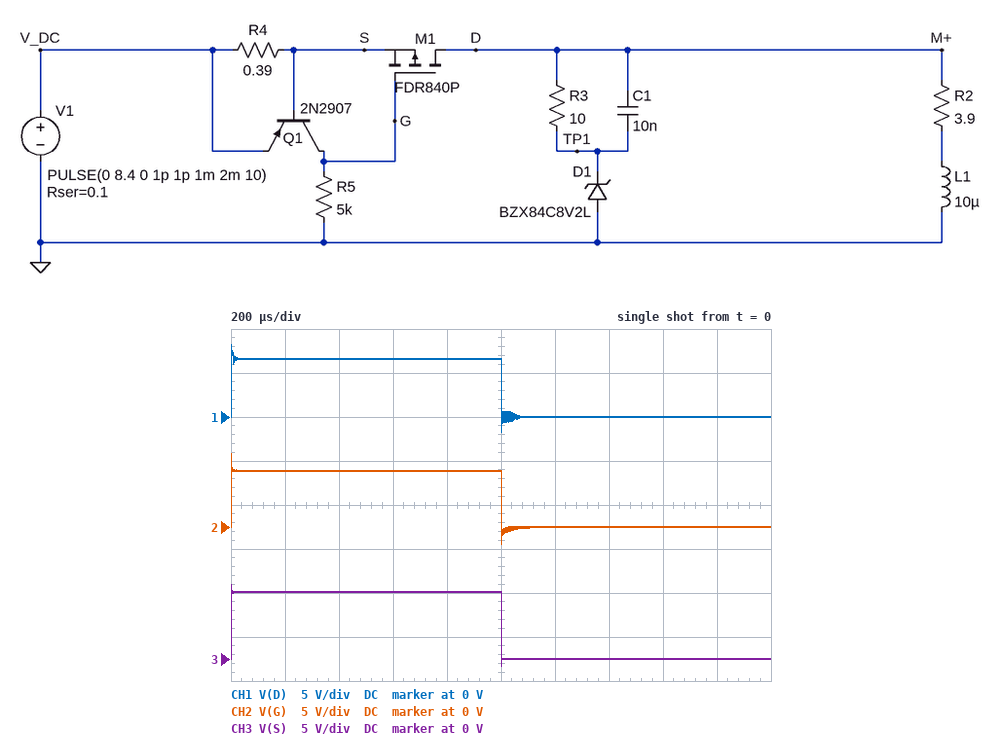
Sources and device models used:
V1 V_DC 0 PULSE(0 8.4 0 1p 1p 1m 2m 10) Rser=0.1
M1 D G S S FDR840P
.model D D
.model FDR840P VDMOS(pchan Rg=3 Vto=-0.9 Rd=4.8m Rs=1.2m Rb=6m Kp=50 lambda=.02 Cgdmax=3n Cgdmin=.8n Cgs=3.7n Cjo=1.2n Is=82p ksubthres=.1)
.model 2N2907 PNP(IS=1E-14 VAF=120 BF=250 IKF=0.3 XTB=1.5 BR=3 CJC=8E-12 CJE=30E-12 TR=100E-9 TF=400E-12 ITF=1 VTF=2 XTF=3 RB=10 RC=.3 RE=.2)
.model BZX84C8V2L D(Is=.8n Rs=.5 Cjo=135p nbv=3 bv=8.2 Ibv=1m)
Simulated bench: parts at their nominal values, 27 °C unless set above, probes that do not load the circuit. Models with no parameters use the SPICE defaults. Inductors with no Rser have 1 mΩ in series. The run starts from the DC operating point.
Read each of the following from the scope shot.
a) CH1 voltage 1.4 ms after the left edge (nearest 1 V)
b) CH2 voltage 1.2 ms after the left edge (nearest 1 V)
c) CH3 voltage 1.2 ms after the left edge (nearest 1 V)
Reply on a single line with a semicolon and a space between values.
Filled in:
0 V; 0 V; 0 V
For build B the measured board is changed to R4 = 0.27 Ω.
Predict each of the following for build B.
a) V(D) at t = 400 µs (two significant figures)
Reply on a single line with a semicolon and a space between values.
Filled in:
7.7 V
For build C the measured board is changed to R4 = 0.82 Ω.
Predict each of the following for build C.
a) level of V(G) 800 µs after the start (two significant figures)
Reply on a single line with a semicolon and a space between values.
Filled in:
6.6 V
